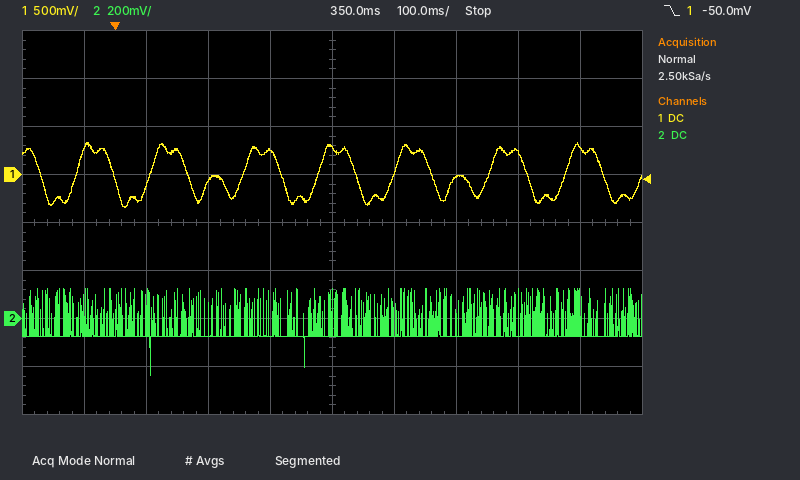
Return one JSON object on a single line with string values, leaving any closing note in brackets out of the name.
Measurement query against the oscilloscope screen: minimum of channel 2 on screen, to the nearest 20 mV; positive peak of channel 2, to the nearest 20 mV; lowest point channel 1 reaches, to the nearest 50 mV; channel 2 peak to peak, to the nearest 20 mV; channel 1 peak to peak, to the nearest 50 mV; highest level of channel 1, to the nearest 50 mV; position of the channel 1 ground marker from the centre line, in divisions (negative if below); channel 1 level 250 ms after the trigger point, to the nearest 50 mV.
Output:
{"minimum of channel 2 on screen, to the nearest 20 mV": "-240 mV", "positive peak of channel 2, to the nearest 20 mV": "120 mV", "lowest point channel 1 reaches, to the nearest 50 mV": "-350 mV", "channel 2 peak to peak, to the nearest 20 mV": "360 mV", "channel 1 peak to peak, to the nearest 50 mV": "700 mV", "highest level of channel 1, to the nearest 50 mV": "350 mV", "position of the channel 1 ground marker from the centre line, in divisions": "+1.0 div", "channel 1 level 250 ms after the trigger point, to the nearest 50 mV": "250 mV"}
